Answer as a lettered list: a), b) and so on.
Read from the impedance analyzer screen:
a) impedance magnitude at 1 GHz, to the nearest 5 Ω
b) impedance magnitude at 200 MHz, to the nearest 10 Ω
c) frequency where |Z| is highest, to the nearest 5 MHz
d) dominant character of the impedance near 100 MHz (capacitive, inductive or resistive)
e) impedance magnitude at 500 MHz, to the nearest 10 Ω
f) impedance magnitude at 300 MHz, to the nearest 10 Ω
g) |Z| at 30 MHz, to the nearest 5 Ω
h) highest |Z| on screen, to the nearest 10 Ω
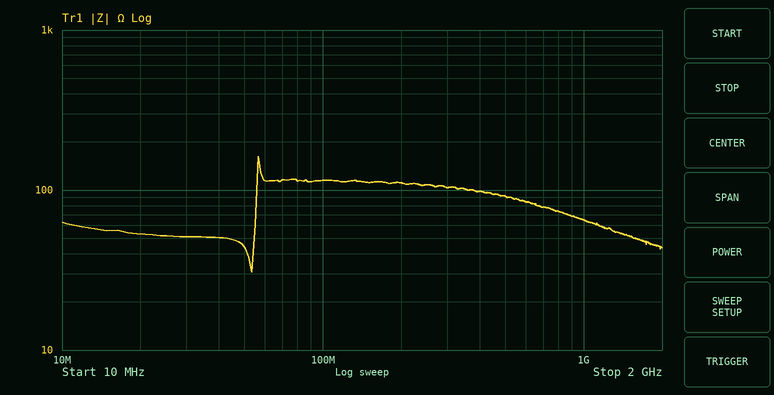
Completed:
a) 65 Ω
b) 110 Ω
c) 55 MHz
d) resistive
e) 90 Ω
f) 100 Ω
g) 50 Ω
h) 160 Ω
